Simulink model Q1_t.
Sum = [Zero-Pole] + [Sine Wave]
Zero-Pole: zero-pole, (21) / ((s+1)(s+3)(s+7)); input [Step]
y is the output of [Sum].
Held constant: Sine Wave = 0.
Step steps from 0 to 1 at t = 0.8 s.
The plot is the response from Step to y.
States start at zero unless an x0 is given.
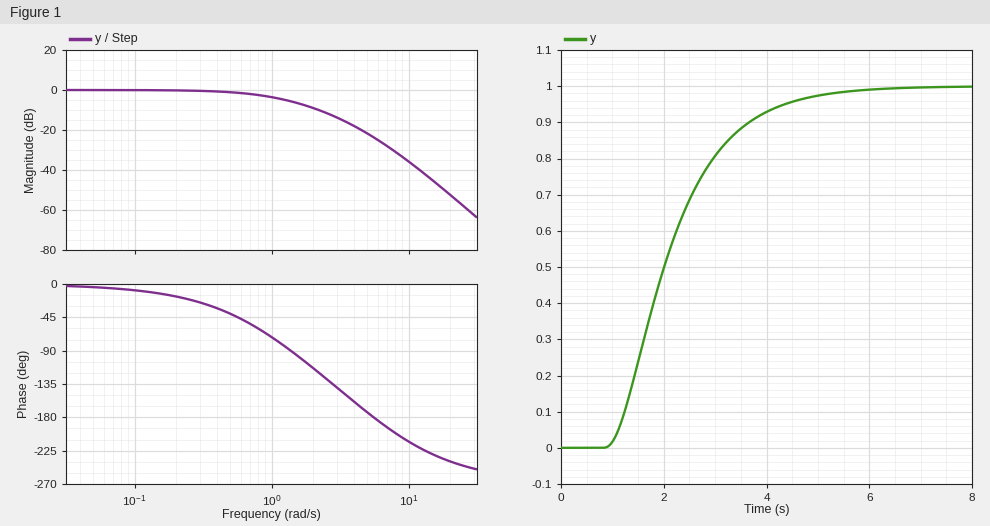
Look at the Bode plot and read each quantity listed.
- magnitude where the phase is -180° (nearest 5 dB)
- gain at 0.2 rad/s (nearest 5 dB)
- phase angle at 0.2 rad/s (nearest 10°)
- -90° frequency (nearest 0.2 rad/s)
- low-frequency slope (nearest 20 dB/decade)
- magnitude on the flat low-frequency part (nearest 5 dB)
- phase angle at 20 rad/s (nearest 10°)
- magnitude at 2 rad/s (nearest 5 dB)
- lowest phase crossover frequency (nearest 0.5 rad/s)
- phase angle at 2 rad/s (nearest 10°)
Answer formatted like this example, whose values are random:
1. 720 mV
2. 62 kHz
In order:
1. -25 dB
2. 0 dB
3. -20°
4. 1.4 rad/s
5. 0 dB/decade
6. 0 dB
7. -240°
8. -10 dB
9. 5.5 rad/s
10. -110°
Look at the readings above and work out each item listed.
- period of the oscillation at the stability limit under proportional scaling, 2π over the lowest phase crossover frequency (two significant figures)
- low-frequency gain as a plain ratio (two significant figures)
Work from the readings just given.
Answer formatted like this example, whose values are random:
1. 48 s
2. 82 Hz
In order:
1. 1.1 s
2. 1.0
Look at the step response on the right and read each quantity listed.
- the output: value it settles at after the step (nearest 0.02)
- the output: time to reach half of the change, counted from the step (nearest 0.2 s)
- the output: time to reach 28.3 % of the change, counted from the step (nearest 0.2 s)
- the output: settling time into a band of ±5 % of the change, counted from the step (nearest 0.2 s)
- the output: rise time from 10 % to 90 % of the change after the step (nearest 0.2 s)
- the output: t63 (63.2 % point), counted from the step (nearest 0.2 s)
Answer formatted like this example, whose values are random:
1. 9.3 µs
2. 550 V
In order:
1. 1.00
2. 1.2 s
3. 0.8 s
4. 3.6 s
5. 2.4 s
6. 1.6 s
